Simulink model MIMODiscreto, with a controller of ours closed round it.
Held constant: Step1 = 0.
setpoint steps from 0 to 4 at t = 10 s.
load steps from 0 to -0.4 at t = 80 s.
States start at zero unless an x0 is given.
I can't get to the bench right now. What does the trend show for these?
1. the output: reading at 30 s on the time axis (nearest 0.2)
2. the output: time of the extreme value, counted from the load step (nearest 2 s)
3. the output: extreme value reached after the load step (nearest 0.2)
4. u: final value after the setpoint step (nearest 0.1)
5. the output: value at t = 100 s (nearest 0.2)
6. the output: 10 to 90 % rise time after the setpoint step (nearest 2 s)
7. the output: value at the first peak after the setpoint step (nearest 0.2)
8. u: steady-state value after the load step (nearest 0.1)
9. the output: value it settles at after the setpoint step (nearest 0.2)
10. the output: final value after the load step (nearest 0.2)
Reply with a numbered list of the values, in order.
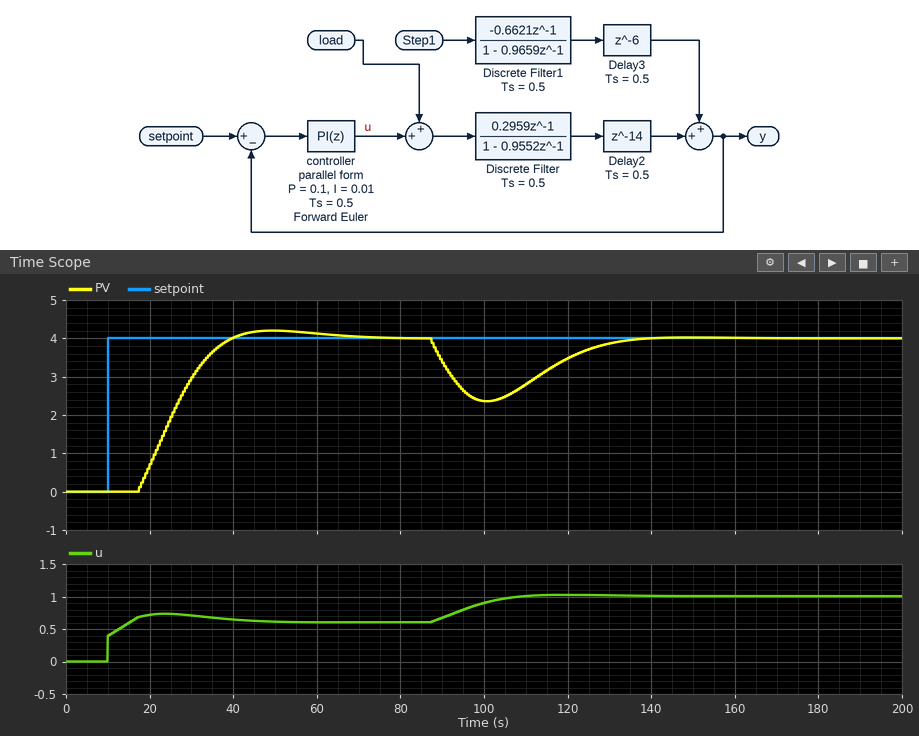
1. 3.0
2. 20 s
3. 2.4
4. 0.6
5. 2.4
6. 16 s
7. 4.2
8. 1.0
9. 4.0
10. 4.0
